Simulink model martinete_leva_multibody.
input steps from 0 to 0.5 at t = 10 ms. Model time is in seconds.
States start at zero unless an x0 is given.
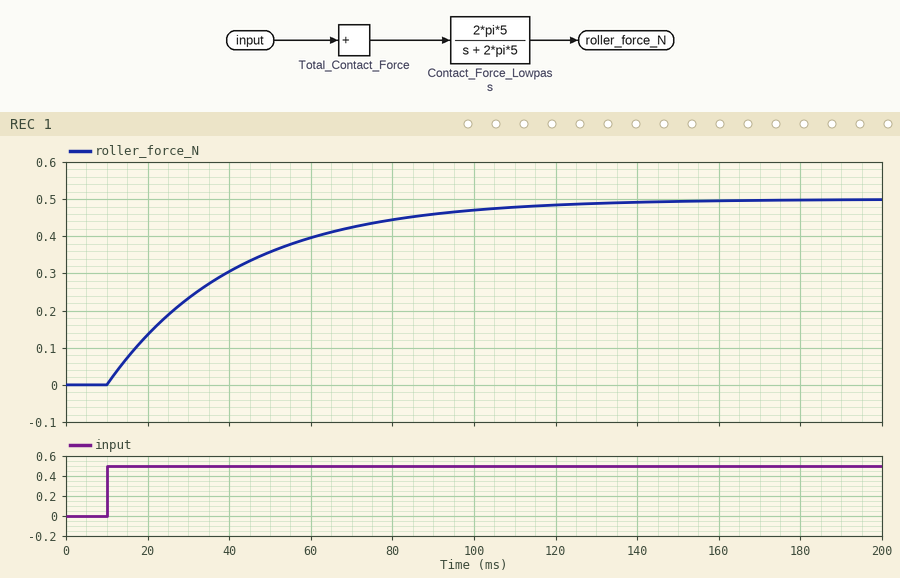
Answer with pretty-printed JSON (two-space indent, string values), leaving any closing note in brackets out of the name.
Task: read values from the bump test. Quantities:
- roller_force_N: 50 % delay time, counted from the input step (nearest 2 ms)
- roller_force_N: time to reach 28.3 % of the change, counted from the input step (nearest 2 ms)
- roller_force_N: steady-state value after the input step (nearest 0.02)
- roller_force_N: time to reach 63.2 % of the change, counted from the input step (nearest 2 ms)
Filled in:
{
  "roller_force_N: 50 % delay time, counted from the input step": "22 ms",
  "roller_force_N: time to reach 28.3 % of the change, counted from the input step": "10 ms",
  "roller_force_N: steady-state value after the input step": "0.50",
  "roller_force_N: time to reach 63.2 % of the change, counted from the input step": "32 ms"
}
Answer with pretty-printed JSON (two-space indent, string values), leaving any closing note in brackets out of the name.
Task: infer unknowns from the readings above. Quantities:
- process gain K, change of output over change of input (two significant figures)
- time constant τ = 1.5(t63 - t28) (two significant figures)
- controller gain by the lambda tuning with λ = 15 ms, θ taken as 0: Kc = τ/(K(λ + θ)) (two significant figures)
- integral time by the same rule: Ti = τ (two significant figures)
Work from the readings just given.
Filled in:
{
  "process gain K, change of output over change of input": "1.0",
  "time constant τ = 1.5(t63 - t28)": "33 ms",
  "controller gain by the lambda tuning with λ = 15 ms, θ taken as 0: Kc = τ/(K(λ + θ))": "2.2",
  "integral time by the same rule: Ti = τ": "33 ms"
}
